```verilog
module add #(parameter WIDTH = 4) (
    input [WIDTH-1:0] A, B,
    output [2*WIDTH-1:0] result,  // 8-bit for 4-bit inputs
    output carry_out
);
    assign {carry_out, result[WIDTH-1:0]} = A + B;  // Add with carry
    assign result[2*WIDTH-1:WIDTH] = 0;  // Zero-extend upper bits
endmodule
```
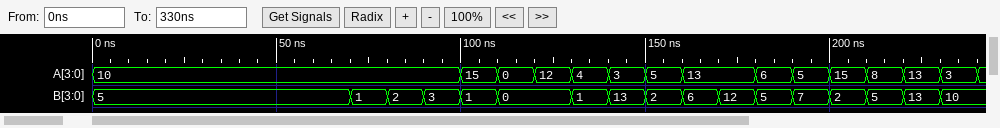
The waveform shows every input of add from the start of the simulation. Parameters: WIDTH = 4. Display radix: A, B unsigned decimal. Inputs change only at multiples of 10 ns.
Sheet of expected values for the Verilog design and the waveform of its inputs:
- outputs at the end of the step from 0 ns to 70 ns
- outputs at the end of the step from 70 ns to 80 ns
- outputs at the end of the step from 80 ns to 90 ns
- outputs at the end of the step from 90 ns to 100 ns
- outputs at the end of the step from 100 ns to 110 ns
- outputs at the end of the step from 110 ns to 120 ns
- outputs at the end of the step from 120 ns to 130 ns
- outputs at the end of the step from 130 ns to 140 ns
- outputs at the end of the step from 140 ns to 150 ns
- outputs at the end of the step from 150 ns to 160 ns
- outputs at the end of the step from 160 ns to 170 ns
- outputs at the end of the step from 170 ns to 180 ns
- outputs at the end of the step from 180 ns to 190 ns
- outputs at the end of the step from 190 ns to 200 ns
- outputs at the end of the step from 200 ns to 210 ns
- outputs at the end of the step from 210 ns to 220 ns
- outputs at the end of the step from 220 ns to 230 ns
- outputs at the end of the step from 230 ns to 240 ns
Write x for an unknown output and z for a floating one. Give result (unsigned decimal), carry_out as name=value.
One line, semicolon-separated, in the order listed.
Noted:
result=15, carry_out=0; result=11, carry_out=0; result=12, carry_out=0; result=13, carry_out=0; result=0, carry_out=1; result=0, carry_out=0; result=12, carry_out=0; result=5, carry_out=0; result=0, carry_out=1; result=7, carry_out=0; result=3, carry_out=1; result=9, carry_out=1; result=11, carry_out=0; result=12, carry_out=0; result=1, carry_out=1; result=13, carry_out=0; result=10, carry_out=1; result=13, carry_out=0
